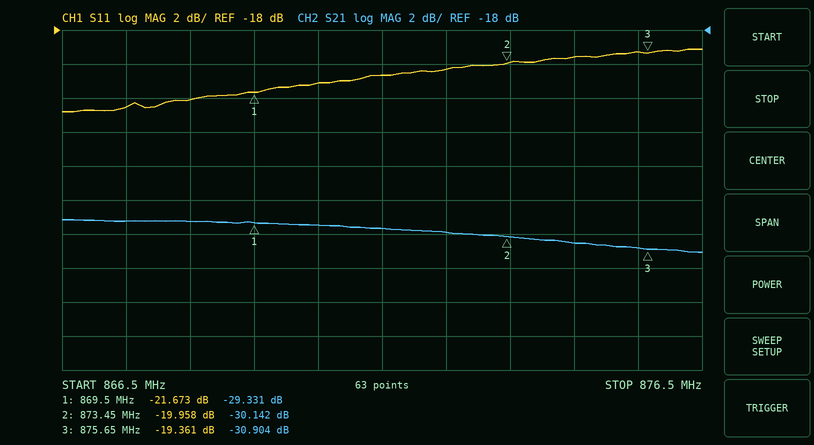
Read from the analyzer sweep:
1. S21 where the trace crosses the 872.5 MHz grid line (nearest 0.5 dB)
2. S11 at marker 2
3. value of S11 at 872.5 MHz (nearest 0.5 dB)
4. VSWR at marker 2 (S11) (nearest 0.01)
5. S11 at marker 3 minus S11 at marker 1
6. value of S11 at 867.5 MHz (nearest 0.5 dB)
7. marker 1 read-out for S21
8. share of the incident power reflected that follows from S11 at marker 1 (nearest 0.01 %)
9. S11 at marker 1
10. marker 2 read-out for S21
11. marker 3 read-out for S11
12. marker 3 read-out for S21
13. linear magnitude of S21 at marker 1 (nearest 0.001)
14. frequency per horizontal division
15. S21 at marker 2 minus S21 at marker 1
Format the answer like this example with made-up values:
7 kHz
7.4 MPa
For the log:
-30.0 dB
-19.958 dB
-20.5 dB
1.22
2.312 dB
-22.5 dB
-29.331 dB
0.68 %
-21.673 dB
-30.142 dB
-19.361 dB
-30.904 dB
0.034
1 MHz
-0.811 dB
